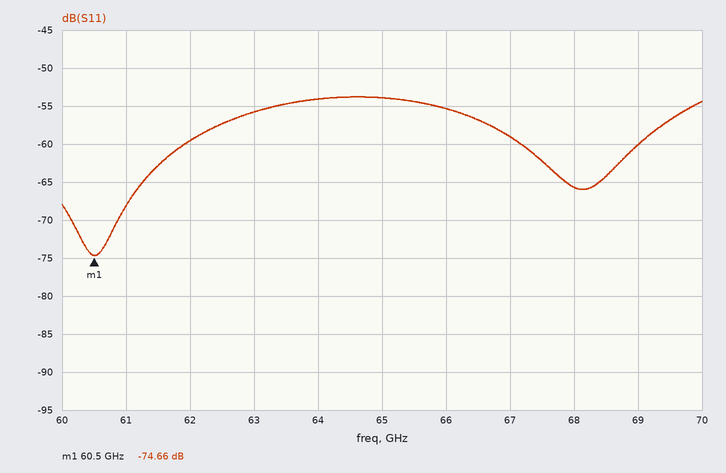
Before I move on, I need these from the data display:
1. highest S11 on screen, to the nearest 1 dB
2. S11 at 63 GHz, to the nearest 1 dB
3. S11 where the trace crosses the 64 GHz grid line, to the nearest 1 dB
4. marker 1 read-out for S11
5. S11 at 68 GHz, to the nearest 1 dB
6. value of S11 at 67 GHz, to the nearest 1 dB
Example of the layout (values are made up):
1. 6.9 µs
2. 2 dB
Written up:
1. -54 dB
2. -56 dB
3. -54 dB
4. -74.66 dB
5. -66 dB
6. -59 dB
